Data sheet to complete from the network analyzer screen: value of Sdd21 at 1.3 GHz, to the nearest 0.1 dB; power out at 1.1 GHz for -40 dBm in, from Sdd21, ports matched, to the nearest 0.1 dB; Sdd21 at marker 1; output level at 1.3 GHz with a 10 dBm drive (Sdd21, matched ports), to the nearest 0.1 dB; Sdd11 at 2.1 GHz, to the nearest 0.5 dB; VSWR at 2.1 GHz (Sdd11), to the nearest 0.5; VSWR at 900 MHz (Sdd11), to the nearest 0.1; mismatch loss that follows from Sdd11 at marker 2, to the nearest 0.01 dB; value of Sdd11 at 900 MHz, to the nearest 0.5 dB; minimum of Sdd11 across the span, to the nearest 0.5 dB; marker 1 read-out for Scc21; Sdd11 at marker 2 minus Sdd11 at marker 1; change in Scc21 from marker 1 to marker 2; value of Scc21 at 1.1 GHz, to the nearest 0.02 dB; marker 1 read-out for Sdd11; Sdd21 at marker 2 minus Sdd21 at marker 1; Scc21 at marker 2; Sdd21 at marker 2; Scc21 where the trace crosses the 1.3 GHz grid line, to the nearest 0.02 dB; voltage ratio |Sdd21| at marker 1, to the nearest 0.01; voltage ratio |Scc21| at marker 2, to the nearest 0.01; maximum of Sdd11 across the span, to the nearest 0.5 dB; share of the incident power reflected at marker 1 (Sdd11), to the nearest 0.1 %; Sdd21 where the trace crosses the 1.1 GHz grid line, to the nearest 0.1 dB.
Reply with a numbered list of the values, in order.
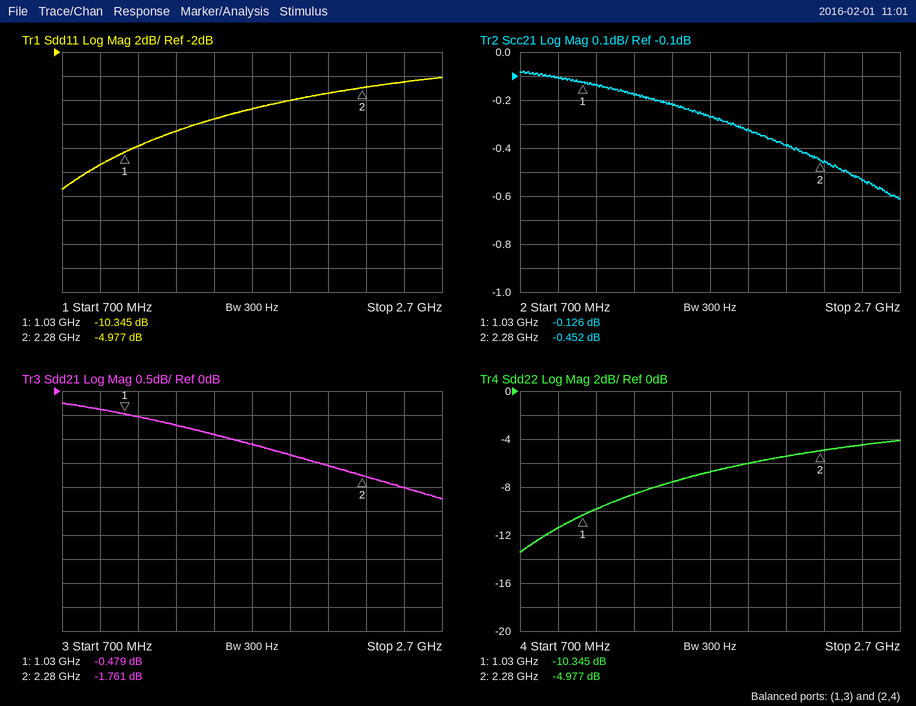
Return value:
1. -0.7 dB
2. -40.5 dBm
3. -0.479 dB
4. 9.3 dBm
5. -5.5 dB
6. 3.5
7. 1.7
8. 1.66 dB
9. -11.5 dB
10. -13.5 dB
11. -0.126 dB
12. 5.368 dB
13. -0.326 dB
14. -0.14 dB
15. -10.345 dB
16. -1.282 dB
17. -0.452 dB
18. -1.761 dB
19. -0.18 dB
20. 0.95
21. 0.95
22. -4.0 dB
23. 9.2 %
24. -0.5 dB
